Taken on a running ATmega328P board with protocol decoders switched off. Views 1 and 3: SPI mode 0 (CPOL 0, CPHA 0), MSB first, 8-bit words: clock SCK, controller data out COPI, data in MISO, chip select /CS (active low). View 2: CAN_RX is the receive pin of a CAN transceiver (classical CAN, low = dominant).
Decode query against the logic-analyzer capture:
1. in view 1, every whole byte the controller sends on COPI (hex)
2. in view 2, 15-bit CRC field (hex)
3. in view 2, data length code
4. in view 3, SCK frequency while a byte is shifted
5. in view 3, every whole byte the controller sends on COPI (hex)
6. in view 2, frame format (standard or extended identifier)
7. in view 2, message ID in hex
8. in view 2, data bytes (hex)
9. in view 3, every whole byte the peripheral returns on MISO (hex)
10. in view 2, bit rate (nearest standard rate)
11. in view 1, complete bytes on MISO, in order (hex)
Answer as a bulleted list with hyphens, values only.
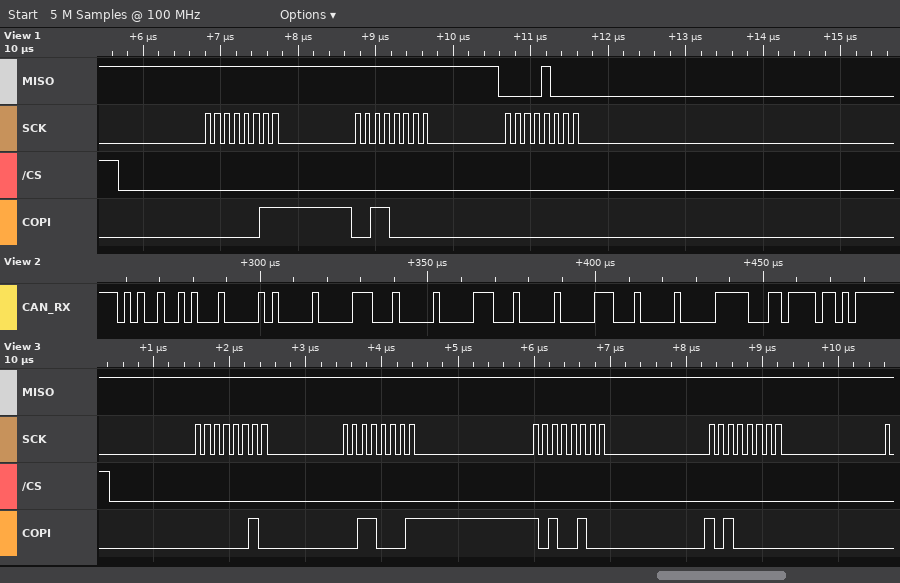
- 03 30 00
- 0x66F6
- 8
- 8 MHz
- 0x02 0x31 0xA4 0xA0
- standard
- 0x525
- 10 03 10 03 10 03 10 03
- 0xFF 0xFF 0xFF 0xFF
- 500 kbit/s
- FF FF 08
